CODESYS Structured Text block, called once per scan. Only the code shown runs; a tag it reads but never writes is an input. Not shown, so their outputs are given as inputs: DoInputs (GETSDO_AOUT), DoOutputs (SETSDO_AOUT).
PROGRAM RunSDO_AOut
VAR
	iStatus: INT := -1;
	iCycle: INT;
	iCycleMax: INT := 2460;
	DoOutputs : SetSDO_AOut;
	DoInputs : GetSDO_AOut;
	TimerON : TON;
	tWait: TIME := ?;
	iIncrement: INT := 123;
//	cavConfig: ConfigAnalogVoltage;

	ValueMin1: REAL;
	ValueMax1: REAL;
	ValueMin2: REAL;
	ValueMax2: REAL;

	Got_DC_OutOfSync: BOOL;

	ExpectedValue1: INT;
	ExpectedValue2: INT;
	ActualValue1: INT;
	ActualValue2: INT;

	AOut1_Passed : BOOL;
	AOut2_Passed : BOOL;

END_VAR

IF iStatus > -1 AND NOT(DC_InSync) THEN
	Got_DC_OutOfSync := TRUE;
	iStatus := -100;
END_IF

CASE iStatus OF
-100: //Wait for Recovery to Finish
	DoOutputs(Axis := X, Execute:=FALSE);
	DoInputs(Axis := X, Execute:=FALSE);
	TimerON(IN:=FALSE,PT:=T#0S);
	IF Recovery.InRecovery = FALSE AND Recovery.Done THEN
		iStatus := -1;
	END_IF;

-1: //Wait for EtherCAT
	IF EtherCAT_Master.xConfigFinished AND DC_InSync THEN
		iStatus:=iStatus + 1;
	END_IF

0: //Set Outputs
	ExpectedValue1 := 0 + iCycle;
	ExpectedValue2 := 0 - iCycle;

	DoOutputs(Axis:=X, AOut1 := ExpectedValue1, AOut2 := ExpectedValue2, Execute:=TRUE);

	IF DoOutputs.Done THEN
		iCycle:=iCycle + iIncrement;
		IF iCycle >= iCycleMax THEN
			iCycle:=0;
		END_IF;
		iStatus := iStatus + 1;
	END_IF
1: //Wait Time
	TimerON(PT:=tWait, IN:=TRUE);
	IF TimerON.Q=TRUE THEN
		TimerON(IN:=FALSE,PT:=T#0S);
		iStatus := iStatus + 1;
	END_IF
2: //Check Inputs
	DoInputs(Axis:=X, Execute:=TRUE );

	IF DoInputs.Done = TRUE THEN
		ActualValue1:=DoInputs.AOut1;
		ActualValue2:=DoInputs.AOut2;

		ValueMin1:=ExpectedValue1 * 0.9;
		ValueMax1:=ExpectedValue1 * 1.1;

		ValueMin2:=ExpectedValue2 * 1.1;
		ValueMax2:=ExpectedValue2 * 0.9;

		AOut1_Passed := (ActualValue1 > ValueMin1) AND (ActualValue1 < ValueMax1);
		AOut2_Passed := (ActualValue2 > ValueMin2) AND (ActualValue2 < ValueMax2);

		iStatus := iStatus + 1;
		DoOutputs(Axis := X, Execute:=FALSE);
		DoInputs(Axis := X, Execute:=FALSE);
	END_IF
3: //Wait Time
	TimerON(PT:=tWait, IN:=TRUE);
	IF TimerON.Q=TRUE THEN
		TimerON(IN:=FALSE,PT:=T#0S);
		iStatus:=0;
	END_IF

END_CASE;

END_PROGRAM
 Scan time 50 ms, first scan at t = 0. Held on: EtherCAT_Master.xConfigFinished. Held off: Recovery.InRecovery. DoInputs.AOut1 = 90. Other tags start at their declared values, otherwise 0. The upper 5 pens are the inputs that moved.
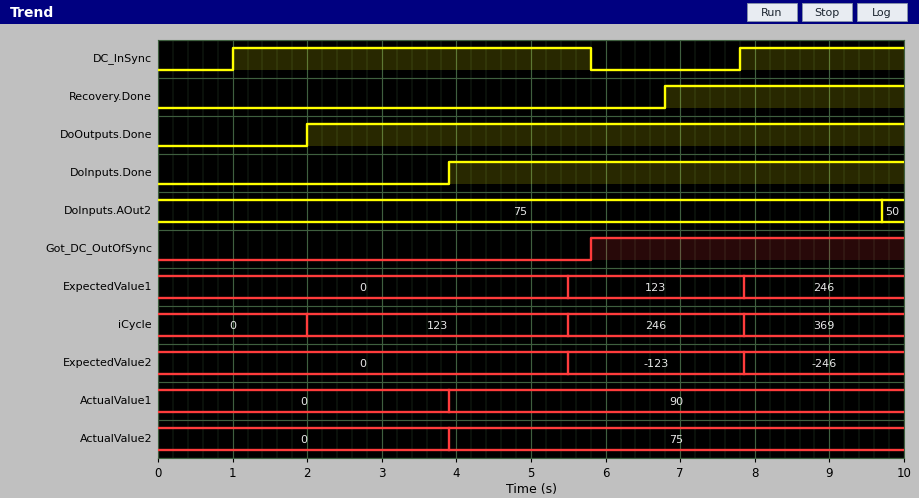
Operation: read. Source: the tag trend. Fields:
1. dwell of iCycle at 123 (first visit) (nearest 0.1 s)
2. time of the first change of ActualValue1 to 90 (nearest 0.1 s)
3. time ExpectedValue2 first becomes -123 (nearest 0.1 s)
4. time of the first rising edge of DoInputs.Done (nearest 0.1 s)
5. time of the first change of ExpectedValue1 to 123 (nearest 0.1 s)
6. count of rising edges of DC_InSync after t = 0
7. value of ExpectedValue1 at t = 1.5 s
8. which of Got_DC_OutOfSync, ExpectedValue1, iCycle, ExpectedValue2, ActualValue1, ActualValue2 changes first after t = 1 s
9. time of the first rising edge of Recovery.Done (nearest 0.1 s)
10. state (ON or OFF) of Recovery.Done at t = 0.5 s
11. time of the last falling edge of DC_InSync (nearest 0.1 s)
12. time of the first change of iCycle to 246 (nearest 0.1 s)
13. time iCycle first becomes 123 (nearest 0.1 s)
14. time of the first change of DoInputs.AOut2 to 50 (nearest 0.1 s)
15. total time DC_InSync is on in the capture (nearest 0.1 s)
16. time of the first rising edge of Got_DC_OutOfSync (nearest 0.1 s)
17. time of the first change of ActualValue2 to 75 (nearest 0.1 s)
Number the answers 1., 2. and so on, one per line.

1. 3.5 s
2. 3.9 s
3. 5.5 s
4. 3.9 s
5. 5.5 s
6. 2
7. 0
8. iCycle
9. 6.8 s
10. OFF
11. 5.8 s
12. 5.5 s
13. 2.0 s
14. 9.7 s
15. 7.0 s
16. 5.8 s
17. 3.9 s
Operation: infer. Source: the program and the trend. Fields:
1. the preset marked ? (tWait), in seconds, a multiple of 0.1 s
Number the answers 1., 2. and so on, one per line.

1. 1.5 s
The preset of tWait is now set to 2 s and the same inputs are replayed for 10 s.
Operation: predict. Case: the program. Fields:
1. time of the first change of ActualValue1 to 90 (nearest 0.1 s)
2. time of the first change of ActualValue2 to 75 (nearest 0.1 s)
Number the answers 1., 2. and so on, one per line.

1. 4.1 s
2. 4.1 s
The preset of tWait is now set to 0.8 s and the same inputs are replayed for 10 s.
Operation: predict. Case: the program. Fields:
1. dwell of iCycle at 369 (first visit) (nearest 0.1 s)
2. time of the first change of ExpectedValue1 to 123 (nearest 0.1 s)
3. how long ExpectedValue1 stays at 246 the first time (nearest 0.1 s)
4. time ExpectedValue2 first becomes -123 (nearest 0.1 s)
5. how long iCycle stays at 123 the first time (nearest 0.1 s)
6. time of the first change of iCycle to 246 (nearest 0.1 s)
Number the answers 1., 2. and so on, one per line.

1. 1.8 s
2. 4.8 s
3. 1.8 s
4. 4.8 s
5. 2.8 s
6. 4.8 s
